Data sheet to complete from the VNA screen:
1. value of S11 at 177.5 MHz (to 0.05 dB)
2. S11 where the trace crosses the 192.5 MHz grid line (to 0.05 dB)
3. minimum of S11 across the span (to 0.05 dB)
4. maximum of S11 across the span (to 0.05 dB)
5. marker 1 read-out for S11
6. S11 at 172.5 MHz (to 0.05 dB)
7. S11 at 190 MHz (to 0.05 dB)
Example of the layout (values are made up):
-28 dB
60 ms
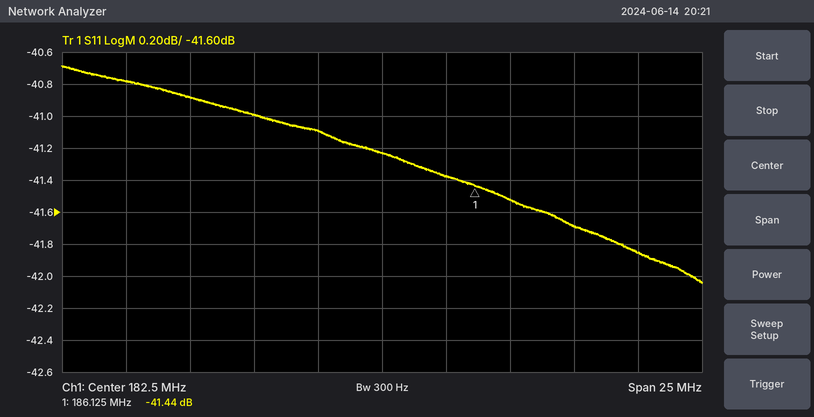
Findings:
-41.00 dB
-41.85 dB
-42.05 dB
-40.70 dB
-41.44 dB
-40.80 dB
-41.70 dB
